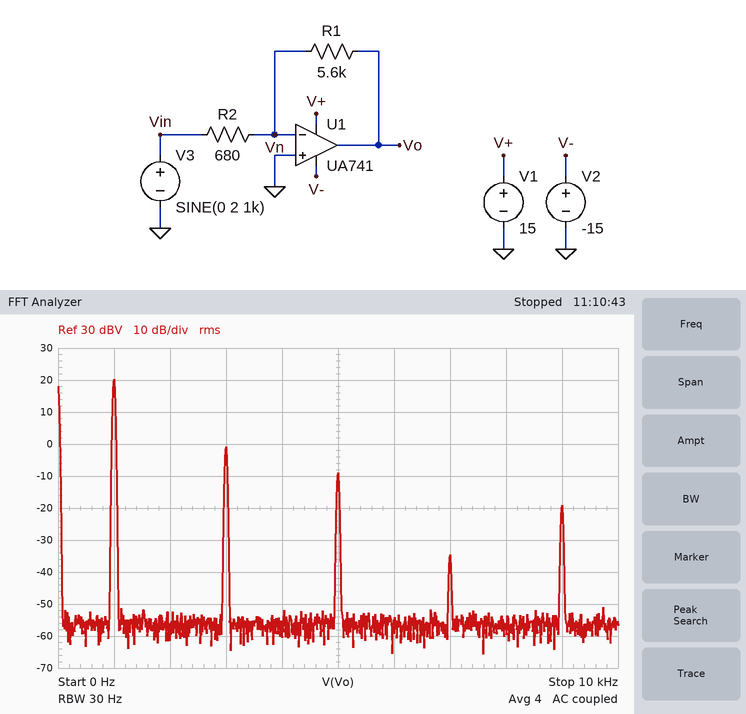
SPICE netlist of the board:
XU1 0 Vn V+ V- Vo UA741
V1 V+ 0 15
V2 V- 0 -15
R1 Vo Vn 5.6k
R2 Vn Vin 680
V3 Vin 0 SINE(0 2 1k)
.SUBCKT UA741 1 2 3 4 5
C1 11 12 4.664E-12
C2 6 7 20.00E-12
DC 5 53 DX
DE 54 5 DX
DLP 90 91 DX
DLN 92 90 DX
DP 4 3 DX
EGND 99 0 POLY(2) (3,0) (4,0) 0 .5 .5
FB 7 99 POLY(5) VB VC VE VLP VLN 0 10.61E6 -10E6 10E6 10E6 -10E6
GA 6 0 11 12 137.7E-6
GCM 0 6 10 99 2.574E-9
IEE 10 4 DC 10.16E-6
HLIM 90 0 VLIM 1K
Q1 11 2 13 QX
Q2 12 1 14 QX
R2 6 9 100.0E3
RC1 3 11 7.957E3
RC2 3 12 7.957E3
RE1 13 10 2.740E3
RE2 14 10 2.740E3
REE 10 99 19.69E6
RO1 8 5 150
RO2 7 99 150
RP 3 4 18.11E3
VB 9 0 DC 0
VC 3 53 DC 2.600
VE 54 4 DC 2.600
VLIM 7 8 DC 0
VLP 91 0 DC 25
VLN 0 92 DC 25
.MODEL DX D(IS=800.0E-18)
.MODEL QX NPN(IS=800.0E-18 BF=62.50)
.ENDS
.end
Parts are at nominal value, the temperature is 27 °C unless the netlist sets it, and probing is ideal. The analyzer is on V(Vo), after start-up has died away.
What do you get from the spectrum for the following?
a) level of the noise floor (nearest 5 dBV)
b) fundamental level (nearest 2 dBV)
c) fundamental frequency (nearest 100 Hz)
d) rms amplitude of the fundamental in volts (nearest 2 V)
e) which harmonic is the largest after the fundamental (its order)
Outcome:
-55 dBV
20 dBV
1.0 kHz
10 V
3
